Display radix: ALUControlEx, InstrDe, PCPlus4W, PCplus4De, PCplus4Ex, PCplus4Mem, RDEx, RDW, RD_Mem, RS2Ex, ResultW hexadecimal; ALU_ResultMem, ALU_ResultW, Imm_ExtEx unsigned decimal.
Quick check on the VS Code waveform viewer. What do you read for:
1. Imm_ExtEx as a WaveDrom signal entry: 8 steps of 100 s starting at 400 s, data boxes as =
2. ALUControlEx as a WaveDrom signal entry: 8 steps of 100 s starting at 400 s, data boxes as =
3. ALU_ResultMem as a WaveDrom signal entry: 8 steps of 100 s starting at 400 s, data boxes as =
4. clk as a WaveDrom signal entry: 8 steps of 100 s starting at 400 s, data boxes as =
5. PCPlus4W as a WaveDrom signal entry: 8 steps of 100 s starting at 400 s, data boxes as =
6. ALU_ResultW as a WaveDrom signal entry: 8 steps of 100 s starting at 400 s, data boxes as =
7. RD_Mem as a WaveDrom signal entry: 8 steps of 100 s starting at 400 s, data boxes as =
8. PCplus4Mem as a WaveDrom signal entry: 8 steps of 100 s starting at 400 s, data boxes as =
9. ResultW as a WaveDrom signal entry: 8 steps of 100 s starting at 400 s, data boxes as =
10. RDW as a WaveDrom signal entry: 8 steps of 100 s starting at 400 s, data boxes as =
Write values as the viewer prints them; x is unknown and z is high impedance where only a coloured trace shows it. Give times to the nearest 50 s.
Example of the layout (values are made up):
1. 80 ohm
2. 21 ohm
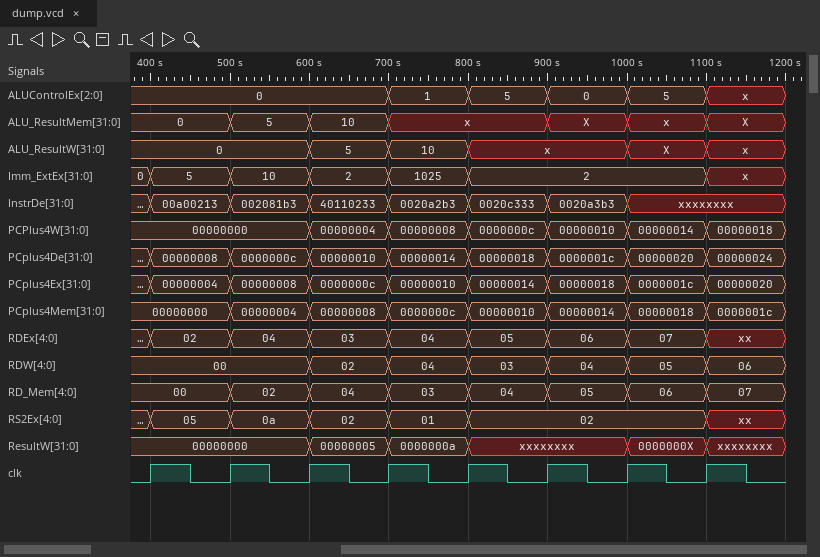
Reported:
1. {name: 'Imm_ExtEx', wave: '=====..x', data: '5 10 2 1025 2'}
2. {name: 'ALUControlEx', wave: '=..====x', data: '0 1 5 0 5'}
3. {name: 'ALU_ResultMem', wave: '===x.=x=', data: '0 5 10 X X'}
4. {name: 'clk', wave: 'p.......'}
5. {name: 'PCPlus4W', wave: '=.======', data: '00000000 00000004 00000008 0000000c 00000010 00000014 00000018'}
6. {name: 'ALU_ResultW', wave: '=.==x.=x', data: '0 5 10 X'}
7. {name: 'RD_Mem', wave: '========', data: '00 02 04 03 04 05 06 07'}
8. {name: 'PCplus4Mem', wave: '========', data: '00000000 00000004 00000008 0000000c 00000010 00000014 00000018 0000001c'}
9. {name: 'ResultW', wave: '=.==x.=x', data: '00000000 00000005 0000000a 0000000X'}
10. {name: 'RDW', wave: '=.======', data: '00 02 04 03 04 05 06'}
